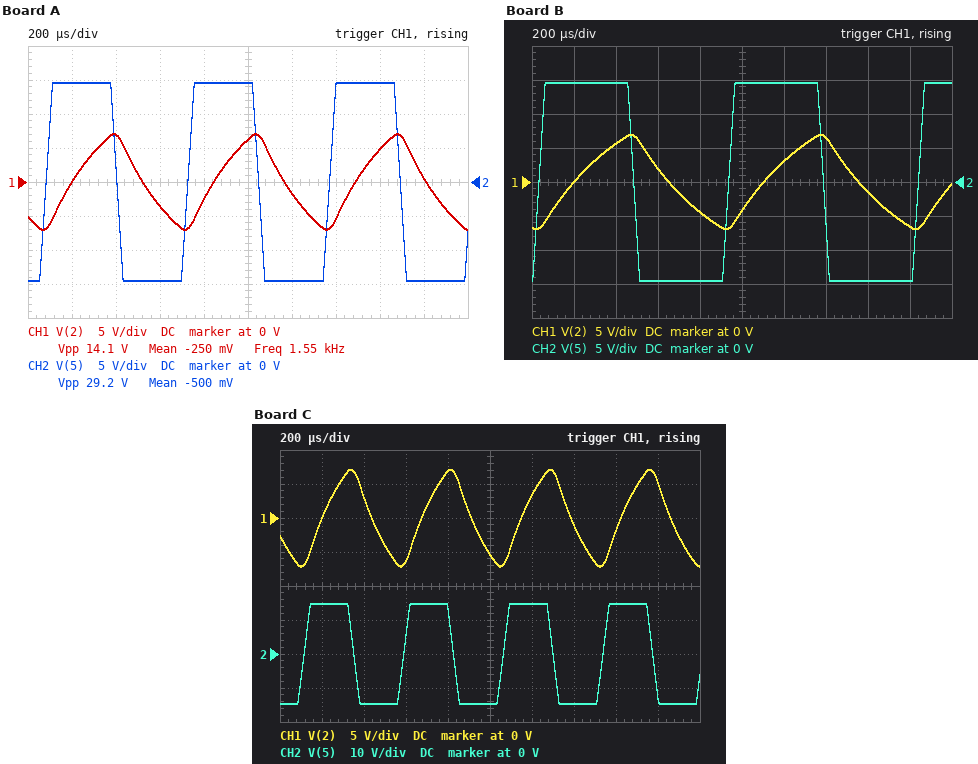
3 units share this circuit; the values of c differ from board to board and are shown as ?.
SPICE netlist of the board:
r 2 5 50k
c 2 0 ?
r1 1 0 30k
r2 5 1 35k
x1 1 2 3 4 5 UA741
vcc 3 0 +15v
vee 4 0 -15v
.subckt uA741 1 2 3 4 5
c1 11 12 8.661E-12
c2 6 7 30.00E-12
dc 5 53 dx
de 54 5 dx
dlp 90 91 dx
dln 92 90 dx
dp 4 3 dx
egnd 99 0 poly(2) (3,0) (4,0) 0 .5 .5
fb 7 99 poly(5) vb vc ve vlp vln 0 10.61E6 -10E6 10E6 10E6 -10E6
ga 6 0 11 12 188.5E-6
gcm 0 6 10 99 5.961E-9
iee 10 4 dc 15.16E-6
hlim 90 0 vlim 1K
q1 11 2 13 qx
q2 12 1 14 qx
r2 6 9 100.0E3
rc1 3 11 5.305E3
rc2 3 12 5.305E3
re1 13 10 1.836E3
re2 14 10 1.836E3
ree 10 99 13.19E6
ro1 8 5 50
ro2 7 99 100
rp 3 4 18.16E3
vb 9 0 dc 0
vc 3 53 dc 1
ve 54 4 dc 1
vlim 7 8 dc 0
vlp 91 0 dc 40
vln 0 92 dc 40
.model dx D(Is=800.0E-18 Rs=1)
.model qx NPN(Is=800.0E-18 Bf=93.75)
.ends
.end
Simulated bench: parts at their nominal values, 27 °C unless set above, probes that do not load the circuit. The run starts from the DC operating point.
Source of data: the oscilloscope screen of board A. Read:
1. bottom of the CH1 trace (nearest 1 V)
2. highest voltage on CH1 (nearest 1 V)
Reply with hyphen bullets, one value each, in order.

- -7 V
- 7 V
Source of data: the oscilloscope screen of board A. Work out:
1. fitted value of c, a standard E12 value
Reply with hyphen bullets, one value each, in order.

- 5.6 nF
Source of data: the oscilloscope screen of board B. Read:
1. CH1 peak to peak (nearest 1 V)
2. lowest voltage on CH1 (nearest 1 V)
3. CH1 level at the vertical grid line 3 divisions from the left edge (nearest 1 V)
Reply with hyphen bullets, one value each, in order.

- 14 V
- -7 V
- 2 V
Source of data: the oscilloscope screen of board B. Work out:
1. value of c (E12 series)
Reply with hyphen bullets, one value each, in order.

- 8.2 nF
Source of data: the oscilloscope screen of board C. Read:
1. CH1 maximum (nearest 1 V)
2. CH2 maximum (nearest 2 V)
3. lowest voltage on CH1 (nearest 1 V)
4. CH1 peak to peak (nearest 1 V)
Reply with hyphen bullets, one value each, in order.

- 7 V
- 14 V
- -7 V
- 14 V
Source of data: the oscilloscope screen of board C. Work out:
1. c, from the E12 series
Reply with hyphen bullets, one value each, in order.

- 3.9 nF
